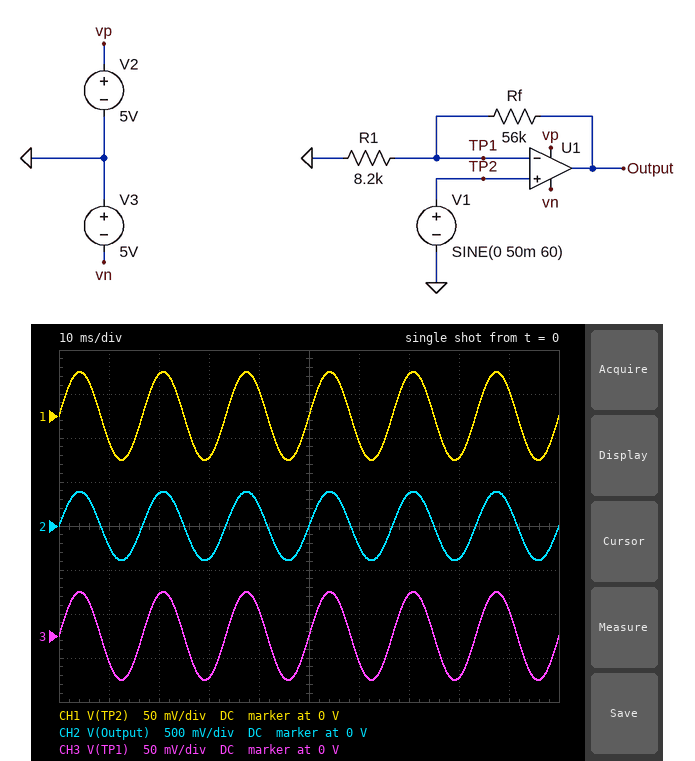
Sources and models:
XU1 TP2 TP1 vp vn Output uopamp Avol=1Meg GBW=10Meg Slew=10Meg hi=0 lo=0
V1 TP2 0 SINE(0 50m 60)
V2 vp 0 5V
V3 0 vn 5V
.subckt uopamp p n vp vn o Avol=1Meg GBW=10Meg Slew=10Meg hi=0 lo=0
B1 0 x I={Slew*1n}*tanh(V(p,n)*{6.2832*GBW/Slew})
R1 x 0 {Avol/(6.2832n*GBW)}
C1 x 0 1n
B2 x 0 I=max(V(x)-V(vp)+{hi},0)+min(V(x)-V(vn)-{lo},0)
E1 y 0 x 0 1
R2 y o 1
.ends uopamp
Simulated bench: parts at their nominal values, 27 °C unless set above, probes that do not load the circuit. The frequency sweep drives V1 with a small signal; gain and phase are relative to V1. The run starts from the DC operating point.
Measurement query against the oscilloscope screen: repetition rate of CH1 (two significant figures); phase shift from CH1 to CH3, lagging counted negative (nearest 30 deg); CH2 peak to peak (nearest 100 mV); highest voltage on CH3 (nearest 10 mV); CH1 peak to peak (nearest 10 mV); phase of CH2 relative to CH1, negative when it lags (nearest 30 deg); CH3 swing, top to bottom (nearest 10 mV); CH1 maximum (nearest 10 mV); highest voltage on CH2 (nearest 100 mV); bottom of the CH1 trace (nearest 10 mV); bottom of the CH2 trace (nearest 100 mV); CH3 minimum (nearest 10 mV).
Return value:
60 Hz
0 deg
800 mV
50 mV
100 mV
0 deg
100 mV
50 mV
400 mV
-50 mV
-400 mV
-50 mV
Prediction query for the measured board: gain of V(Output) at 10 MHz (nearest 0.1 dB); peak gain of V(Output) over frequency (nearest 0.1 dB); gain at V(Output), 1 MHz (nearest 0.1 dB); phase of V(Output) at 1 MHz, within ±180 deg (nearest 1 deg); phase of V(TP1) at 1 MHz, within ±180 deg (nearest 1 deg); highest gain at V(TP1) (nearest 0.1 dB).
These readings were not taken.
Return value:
-0.1 dB
17.9 dB
15.8 dB
-38 deg
-38 deg
0 dB
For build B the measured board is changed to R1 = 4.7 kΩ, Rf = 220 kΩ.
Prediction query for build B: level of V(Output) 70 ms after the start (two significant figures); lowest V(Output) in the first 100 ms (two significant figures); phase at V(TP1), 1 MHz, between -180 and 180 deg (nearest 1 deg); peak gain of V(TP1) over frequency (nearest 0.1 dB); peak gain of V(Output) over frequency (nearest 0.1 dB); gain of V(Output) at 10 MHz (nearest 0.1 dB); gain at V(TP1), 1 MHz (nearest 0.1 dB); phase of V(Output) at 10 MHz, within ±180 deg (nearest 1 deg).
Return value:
2.3 V
-2.4 V
-78 deg
0 dB
33.6 dB
0 dB
-13.8 dB
-89 deg
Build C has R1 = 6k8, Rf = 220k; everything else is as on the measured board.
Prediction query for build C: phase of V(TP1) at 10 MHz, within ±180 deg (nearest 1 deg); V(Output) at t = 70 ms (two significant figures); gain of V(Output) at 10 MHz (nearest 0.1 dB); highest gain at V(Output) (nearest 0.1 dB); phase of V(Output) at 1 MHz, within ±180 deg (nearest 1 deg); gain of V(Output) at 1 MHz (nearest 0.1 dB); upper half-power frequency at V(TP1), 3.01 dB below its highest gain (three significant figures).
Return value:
-88 deg
1.6 V
0 dB
30.5 dB
-73 deg
19.6 dB
300 kHz
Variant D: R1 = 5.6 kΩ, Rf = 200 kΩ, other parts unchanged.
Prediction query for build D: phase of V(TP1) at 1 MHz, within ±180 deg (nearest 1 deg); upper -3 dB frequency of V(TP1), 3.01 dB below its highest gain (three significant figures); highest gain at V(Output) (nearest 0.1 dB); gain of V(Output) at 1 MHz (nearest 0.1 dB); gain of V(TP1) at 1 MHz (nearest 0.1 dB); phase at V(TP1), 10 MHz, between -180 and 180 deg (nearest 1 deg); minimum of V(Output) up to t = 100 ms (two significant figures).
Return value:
-75 deg
272 kHz
31.3 dB
19.7 dB
-11.6 dB
-88 deg
-1.8 V
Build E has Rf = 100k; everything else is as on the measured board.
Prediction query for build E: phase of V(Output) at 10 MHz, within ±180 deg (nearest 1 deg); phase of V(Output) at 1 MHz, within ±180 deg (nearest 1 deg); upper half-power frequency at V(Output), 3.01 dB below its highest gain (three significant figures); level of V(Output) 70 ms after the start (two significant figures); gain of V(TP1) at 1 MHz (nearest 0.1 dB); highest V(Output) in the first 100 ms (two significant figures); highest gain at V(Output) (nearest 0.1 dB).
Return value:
-86 deg
-53 deg
758 kHz
630 mV
-4.4 dB
660 mV
22.4 dB
